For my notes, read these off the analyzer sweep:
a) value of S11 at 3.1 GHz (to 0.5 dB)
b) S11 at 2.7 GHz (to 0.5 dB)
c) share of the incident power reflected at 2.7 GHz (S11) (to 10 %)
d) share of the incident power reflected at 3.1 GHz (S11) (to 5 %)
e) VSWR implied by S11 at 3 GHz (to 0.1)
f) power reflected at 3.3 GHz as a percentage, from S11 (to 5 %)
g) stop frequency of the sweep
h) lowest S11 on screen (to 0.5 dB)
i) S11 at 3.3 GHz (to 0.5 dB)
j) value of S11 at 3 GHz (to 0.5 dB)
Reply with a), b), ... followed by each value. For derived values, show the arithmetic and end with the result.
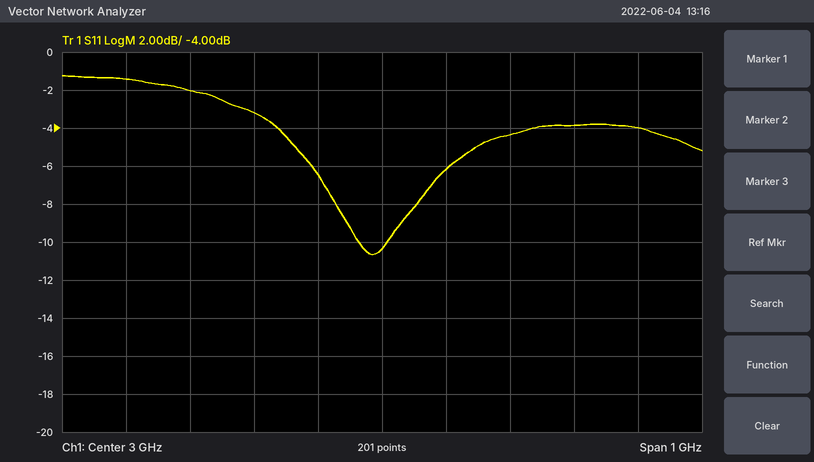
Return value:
a) -6.0 dB
b) -2.0 dB
c) 10^(-2/10) ≈ 63.1 %, so 60 % to the nearest 10 %
d) 10^(-6/10) ≈ 25 %
e) |Γ| = 10^(-10.5/20) = 0.2985; VSWR = (1 + 0.2985)/(1 − 0.2985) ≈ 1.9
f) 10^(-4/10) ≈ 40 %
g) 3.5 GHz
h) -10.5 dB
i) -4.0 dB
j) -10.5 dB
